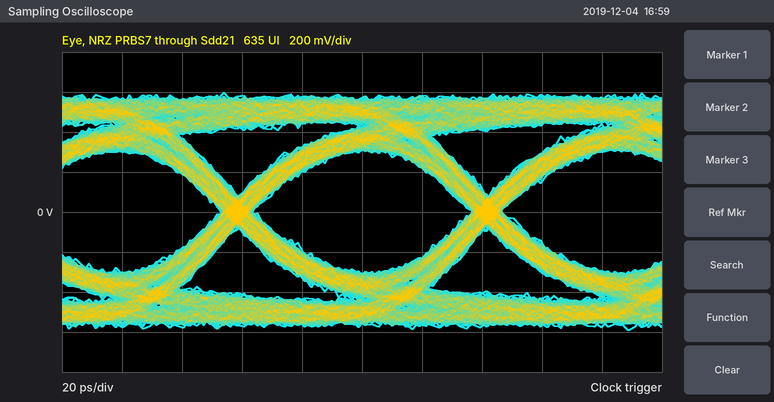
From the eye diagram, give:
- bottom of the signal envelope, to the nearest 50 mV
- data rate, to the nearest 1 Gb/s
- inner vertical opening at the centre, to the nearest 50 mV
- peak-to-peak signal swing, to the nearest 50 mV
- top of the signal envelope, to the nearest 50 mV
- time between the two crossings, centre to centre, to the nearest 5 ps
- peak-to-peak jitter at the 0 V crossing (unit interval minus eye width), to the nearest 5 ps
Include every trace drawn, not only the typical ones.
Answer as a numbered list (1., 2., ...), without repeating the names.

1. -600 mV
2. 12 Gb/s
3. 600 mV
4. 1.20 V
5. 600 mV
6. 85 ps
7. 10 ps
